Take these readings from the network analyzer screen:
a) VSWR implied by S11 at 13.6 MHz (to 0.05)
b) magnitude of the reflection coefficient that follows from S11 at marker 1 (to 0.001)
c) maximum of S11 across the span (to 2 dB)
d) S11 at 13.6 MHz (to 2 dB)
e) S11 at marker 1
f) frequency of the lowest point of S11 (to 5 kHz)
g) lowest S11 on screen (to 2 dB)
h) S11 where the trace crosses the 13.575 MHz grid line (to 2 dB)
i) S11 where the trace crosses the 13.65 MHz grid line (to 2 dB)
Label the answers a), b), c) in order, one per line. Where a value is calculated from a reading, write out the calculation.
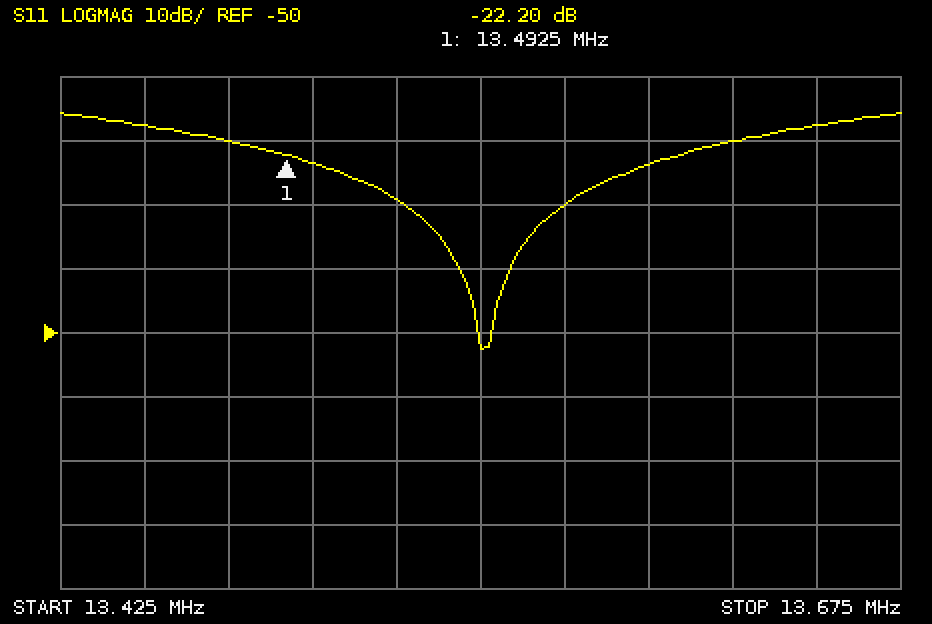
a) |Γ| = 10^(-24/20) = 0.0631; VSWR = (1 + 0.0631)/(1 − 0.0631) ≈ 1.13, so 1.15 to the nearest 0.05
b) 10^(-22.2/20) ≈ 0.078
c) -16 dB
d) -24 dB
e) -22.20 dB
f) 13.550 MHz
g) -52 dB
h) -30 dB
i) -18 dB
